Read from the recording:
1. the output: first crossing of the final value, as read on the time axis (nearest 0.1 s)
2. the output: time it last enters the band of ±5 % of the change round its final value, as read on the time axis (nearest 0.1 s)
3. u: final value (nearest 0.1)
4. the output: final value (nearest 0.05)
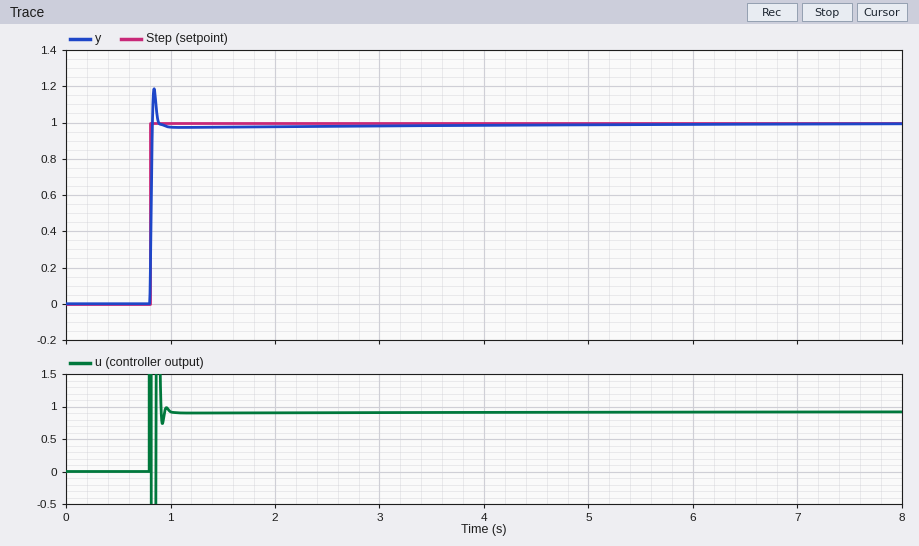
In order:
0.8 s
0.9 s
0.9
1.00
